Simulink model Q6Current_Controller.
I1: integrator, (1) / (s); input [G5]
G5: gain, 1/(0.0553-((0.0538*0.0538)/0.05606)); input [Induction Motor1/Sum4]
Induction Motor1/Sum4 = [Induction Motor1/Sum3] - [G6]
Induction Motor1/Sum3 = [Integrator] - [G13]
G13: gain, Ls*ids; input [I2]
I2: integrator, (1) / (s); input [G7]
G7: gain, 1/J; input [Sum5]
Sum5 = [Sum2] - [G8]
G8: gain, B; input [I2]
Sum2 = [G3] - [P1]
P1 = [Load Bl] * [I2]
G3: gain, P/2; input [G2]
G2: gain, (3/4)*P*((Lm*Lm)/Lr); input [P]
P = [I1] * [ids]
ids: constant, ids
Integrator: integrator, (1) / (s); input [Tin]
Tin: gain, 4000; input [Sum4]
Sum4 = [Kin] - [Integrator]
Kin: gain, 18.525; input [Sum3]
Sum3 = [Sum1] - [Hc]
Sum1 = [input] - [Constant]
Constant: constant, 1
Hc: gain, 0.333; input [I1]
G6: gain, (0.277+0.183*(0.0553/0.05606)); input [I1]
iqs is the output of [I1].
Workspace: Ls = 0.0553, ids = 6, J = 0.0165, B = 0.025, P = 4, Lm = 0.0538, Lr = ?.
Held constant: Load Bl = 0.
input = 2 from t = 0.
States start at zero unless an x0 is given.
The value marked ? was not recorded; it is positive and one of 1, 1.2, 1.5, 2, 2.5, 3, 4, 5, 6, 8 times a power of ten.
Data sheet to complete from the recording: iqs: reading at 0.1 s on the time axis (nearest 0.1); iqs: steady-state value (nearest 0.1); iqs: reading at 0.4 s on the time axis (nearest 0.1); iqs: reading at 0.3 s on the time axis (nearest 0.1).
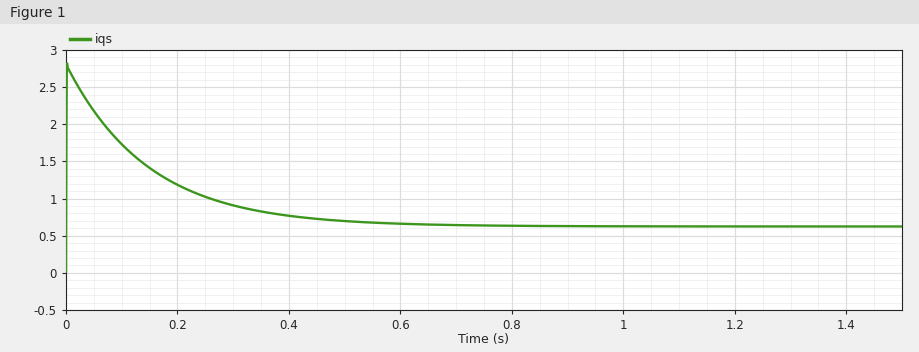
1.7
0.6
0.8
0.9
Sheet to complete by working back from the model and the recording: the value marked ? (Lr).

0.06
